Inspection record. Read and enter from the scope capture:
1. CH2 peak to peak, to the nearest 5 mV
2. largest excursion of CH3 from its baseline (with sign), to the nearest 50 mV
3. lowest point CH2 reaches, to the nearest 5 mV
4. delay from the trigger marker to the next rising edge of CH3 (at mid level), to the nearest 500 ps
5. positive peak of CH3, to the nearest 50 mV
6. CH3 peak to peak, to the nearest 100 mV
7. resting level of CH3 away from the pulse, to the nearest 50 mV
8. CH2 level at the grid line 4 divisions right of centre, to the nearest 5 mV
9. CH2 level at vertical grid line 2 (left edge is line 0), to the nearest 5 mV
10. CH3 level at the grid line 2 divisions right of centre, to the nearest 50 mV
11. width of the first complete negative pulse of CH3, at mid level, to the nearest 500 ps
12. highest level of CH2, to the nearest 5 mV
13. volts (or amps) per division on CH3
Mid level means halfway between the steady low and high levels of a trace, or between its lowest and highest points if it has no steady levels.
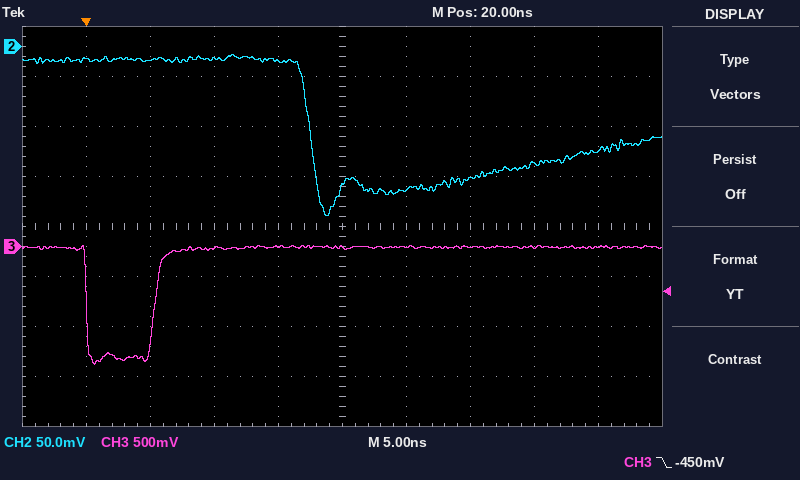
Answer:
160 mV
-1.15 V
-170 mV
5.5 ns
0 mV
1.20 V
0 mV
-105 mV
-15 mV
0 mV
5.5 ns
-10 mV
500 mV
